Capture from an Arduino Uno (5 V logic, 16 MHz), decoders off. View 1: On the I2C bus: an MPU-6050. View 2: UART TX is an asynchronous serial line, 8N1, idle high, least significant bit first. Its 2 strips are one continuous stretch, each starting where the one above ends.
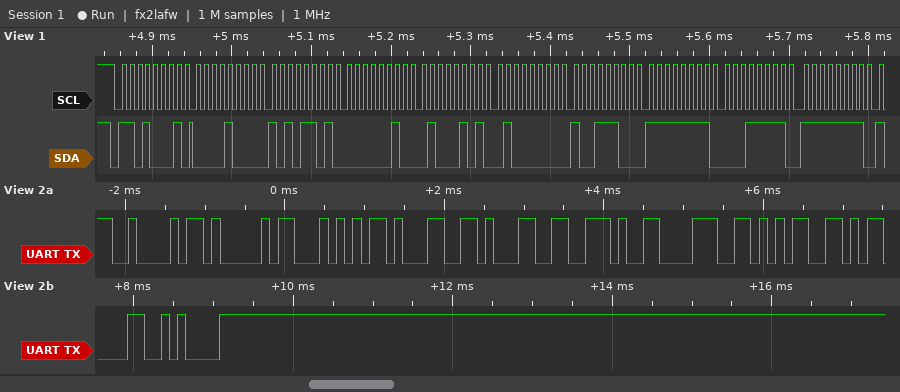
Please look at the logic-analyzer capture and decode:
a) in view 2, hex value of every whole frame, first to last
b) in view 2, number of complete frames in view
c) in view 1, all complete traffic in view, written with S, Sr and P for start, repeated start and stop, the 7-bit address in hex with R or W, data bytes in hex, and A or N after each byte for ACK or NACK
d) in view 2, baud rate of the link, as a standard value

42 41 54 31 31 2E 38 35 0D 0A
10
S 68R A 08 A AD A 02 A 45 A 40 A 9C A FF A 1F A FF A
9600 baud
